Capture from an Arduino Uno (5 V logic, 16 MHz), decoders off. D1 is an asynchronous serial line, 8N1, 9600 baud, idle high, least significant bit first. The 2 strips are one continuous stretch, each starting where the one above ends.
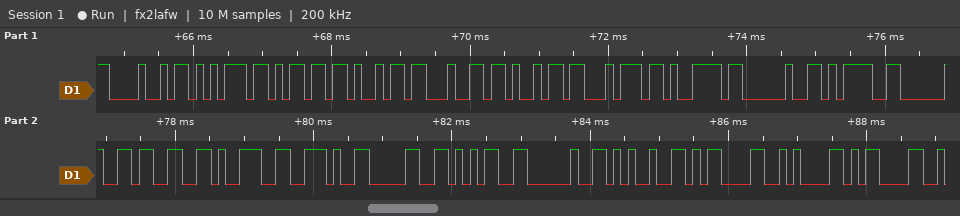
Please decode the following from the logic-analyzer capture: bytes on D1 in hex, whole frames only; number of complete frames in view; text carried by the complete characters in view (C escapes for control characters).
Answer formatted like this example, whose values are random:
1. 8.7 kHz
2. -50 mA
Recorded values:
1. 0x48 0x75 0x6D 0x69 0x64 0x69 0x74 0x79 0x20 0x3D 0x20 0x33 0x39 0x2E 0x30 0x35 0x20 0x25 0x0D 0x0A 0x0D
2. 21
3. "Humidity = 39.05 %\r\n\r"
